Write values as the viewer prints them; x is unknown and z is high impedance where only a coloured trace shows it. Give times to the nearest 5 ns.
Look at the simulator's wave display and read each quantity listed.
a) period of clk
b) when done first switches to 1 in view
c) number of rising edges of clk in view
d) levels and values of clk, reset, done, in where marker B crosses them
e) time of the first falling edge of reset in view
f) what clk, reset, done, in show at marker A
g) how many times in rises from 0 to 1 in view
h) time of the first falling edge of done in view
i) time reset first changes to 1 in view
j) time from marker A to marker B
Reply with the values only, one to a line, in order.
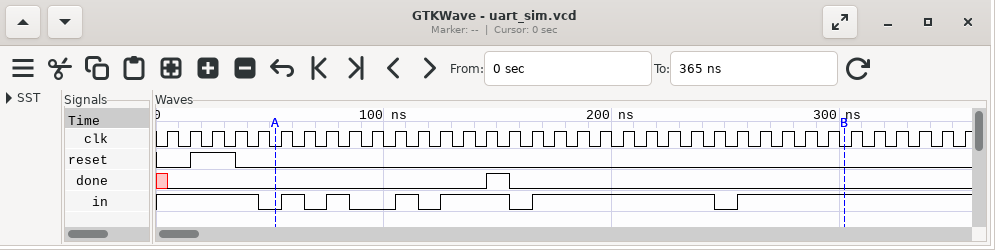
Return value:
10 ns
145 ns
36
clk=0, reset=0, done=0, in=1
35 ns
clk=0, reset=0, done=0, in=0
6
155 ns
15 ns
250 ns
